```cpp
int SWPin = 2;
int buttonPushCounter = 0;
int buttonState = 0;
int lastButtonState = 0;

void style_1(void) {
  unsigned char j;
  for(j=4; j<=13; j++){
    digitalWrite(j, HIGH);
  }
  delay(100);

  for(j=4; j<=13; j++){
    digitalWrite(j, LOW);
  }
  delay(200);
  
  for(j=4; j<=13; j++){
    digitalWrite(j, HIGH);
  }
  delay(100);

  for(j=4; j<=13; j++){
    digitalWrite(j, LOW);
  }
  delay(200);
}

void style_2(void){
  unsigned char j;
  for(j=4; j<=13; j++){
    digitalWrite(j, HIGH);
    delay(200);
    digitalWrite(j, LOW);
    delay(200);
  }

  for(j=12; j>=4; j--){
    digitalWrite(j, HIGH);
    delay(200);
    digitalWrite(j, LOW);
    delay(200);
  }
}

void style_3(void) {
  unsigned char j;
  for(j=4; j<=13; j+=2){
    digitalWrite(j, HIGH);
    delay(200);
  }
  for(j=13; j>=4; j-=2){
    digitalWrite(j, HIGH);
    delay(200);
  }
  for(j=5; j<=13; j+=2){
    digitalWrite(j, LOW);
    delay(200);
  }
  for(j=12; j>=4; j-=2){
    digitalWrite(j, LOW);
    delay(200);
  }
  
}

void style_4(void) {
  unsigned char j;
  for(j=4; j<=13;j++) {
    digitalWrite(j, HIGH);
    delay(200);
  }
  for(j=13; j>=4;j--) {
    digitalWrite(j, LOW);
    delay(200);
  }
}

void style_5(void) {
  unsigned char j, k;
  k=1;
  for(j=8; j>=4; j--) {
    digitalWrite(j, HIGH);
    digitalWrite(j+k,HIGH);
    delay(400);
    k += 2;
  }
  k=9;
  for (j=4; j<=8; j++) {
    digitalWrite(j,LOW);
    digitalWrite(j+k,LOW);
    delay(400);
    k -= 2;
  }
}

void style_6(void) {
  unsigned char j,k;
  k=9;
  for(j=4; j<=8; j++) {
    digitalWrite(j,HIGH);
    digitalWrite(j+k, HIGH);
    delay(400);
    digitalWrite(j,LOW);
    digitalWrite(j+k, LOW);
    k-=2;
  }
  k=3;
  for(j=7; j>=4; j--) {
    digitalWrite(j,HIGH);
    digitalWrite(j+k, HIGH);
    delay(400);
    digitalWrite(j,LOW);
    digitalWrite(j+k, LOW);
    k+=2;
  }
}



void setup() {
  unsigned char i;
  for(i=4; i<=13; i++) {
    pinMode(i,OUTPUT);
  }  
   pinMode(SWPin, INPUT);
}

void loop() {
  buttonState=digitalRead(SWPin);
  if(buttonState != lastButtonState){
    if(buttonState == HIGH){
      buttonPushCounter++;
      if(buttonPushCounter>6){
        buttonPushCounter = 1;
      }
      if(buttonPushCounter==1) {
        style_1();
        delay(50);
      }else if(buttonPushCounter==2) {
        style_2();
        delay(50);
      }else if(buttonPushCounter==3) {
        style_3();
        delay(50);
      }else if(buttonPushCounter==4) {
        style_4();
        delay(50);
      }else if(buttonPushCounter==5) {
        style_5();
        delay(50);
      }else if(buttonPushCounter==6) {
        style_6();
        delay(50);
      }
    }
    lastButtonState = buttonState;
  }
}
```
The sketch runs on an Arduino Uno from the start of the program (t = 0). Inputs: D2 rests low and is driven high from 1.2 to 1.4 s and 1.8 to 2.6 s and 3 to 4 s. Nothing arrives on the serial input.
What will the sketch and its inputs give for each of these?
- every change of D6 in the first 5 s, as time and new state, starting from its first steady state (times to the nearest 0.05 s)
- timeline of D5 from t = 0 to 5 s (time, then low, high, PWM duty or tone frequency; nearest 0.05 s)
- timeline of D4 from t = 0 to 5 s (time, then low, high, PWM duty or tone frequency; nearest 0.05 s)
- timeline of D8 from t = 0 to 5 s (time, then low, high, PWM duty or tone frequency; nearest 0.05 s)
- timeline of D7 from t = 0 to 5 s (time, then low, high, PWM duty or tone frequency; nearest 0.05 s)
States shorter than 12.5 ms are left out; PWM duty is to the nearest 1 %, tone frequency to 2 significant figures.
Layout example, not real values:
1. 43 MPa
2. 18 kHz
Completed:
1. 0 s low; 1.2 s high; 1.3 s low; 1.5 s high; 1.6 s low; 3.8 s high; 4 s low
2. 0 s low; 1.2 s high; 1.3 s low; 1.5 s high; 1.6 s low; 3.4 s high; 3.6 s low
3. 0 s low; 1.2 s high; 1.3 s low; 1.5 s high; 1.6 s low; 3 s high; 3.2 s low
4. 0 s low; 1.2 s high; 1.3 s low; 1.5 s high; 1.6 s low; 4.6 s high; 4.8 s low
5. 0 s low; 1.2 s high; 1.3 s low; 1.5 s high; 1.6 s low; 4.2 s high; 4.4 s low
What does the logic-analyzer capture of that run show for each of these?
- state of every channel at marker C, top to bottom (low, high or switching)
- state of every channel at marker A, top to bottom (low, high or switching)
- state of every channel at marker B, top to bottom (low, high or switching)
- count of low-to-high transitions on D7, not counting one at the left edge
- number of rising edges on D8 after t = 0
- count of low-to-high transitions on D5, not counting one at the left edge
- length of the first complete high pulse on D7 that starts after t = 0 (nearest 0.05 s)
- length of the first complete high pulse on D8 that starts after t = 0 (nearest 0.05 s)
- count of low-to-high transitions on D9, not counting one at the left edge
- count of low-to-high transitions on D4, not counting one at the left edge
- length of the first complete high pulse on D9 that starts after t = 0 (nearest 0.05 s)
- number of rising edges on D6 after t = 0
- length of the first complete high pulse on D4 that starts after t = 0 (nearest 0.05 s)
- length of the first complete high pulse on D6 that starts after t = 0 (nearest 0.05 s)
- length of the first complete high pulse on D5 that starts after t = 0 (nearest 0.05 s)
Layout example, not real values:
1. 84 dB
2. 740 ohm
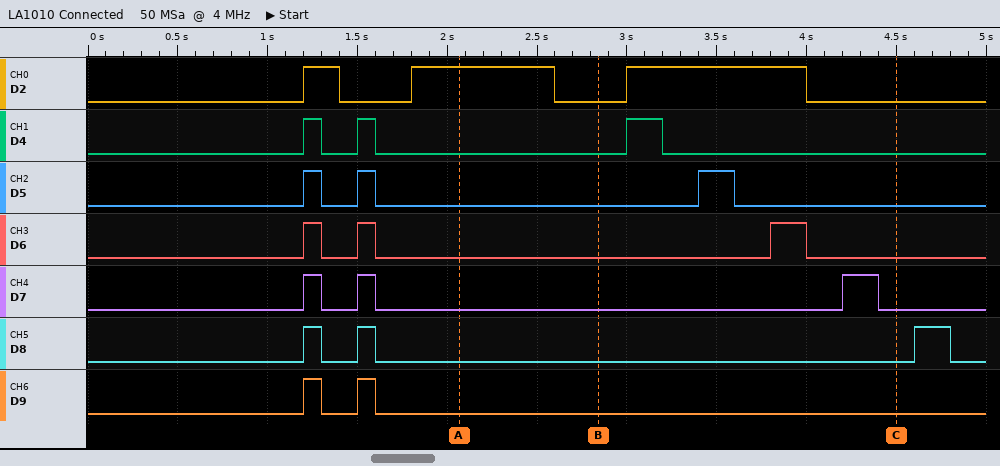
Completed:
1. D2 low, D4 low, D5 low, D6 low, D7 low, D8 low, D9 low
2. D2 high, D4 low, D5 low, D6 low, D7 low, D8 low, D9 low
3. D2 low, D4 low, D5 low, D6 low, D7 low, D8 low, D9 low
4. 3
5. 3
6. 3
7. 0.10 s
8. 0.10 s
9. 2
10. 3
11. 0.10 s
12. 3
13. 0.10 s
14. 0.10 s
15. 0.10 s
